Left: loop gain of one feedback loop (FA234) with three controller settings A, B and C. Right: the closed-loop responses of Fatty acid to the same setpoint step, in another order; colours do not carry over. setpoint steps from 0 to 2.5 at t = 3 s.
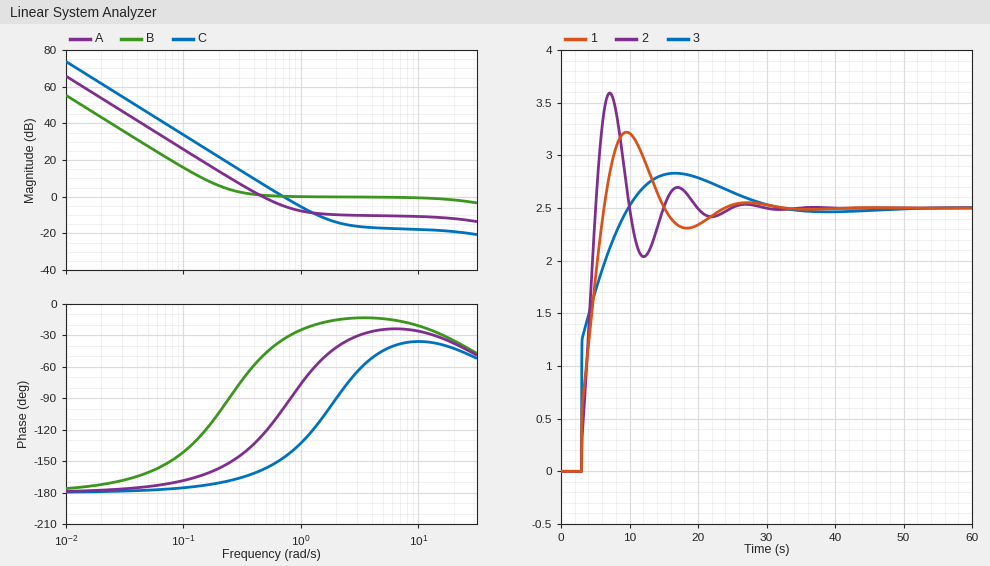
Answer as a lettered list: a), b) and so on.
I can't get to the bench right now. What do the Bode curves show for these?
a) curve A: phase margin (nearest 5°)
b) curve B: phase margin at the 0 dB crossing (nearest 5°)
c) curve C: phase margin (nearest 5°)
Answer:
a) 55°
b) 155°
c) 35°
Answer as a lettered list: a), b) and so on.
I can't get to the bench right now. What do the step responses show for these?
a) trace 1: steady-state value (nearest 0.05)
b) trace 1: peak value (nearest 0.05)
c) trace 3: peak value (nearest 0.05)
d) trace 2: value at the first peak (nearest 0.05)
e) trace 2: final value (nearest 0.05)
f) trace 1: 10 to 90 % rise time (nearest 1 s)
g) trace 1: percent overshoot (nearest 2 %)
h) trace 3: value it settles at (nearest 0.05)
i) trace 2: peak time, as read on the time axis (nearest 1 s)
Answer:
a) 2.50
b) 3.20
c) 2.85
d) 3.60
e) 2.50
f) 3 s
g) 28 %
h) 2.50
i) 7 s
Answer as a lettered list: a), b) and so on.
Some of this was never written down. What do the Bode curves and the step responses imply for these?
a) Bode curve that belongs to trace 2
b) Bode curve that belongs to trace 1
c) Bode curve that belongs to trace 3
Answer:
a) C
b) A
c) B
